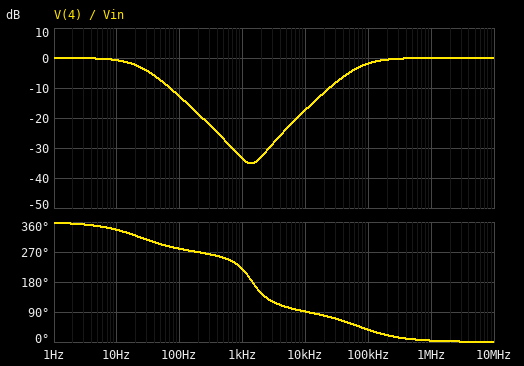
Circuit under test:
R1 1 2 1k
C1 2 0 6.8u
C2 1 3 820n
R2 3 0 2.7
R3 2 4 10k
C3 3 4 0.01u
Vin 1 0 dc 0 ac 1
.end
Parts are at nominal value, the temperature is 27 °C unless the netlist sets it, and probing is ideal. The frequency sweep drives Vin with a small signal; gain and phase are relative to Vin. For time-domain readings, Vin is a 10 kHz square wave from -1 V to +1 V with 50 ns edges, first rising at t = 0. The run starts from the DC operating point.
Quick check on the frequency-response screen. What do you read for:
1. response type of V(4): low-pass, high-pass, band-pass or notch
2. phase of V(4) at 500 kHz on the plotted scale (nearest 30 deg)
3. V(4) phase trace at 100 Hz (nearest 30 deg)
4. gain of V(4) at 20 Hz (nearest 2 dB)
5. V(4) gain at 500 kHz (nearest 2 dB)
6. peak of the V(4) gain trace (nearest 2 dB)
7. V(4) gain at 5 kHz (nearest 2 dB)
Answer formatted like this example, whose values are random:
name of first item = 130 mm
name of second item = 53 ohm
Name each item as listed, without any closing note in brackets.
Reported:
response type of V(4): low-pass, high-pass, band-pass or notch = notch
phase of V(4) at 500 kHz on the plotted scale = 0 deg
V(4) phase trace at 100 Hz = 270 deg
gain of V(4) at 20 Hz = -2 dB
V(4) gain at 500 kHz = 0 dB
peak of the V(4) gain trace = 0 dB
V(4) gain at 5 kHz = -24 dB
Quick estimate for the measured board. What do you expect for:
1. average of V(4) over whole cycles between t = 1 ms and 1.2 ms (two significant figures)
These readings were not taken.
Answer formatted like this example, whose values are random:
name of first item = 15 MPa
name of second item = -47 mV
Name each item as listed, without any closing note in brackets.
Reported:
average of V(4) over whole cycles between t = 1 ms and 1.2 ms = -860 mV
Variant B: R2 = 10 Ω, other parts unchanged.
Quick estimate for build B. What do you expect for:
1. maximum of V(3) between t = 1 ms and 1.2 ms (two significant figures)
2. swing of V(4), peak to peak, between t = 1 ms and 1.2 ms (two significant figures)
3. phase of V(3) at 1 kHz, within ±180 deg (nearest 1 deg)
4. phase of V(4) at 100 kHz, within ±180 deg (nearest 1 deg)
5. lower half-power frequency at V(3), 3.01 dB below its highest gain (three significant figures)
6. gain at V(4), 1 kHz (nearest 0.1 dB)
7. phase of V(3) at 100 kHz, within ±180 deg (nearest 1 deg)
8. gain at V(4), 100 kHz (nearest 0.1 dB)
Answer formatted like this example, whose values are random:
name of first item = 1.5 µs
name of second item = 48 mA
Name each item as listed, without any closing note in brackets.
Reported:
maximum of V(3) between t = 1 ms and 1.2 ms = 2.0 V
swing of V(4), peak to peak, between t = 1 ms and 1.2 ms = 4.1 V
phase of V(3) at 1 kHz, within ±180 deg = 87 deg
phase of V(4) at 100 kHz, within ±180 deg = 12 deg
lower half-power frequency at V(3), 3.01 dB below its highest gain = 19.4 kHz
gain at V(4), 1 kHz = -29.8 dB
phase of V(3) at 100 kHz, within ±180 deg = 11 deg
gain at V(4), 100 kHz = -0.2 dB
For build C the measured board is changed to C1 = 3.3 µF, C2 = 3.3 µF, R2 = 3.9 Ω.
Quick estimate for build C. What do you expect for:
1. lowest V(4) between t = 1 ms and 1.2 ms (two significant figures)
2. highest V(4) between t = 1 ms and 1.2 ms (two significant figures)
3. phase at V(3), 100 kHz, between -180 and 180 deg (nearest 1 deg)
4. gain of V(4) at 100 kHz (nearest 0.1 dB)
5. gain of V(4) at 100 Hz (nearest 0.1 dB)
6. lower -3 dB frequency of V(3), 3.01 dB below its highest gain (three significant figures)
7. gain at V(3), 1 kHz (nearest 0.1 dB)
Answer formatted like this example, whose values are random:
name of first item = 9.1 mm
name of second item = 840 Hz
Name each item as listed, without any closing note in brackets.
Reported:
lowest V(4) between t = 1 ms and 1.2 ms = -2.8 V
highest V(4) between t = 1 ms and 1.2 ms = 1.3 V
phase at V(3), 100 kHz, between -180 and 180 deg = 7 deg
gain of V(4) at 100 kHz = -0.1 dB
gain of V(4) at 100 Hz = -7.3 dB
lower -3 dB frequency of V(3), 3.01 dB below its highest gain = 12.4 kHz
gain at V(3), 1 kHz = -21.9 dB
